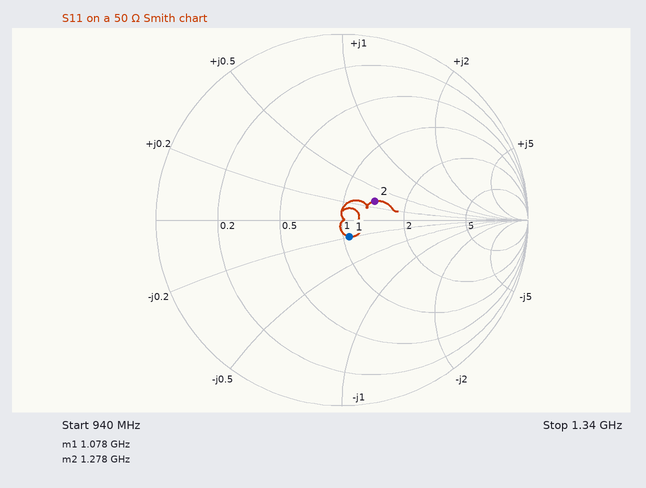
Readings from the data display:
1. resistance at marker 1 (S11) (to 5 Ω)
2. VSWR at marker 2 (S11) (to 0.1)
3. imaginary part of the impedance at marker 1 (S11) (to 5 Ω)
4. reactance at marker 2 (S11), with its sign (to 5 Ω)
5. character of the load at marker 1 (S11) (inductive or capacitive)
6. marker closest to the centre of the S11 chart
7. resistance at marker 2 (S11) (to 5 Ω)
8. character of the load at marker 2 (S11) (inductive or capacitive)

55 Ω
1.5
-10 Ω
+15 Ω
capacitive
marker 1
70 Ω
inductive
